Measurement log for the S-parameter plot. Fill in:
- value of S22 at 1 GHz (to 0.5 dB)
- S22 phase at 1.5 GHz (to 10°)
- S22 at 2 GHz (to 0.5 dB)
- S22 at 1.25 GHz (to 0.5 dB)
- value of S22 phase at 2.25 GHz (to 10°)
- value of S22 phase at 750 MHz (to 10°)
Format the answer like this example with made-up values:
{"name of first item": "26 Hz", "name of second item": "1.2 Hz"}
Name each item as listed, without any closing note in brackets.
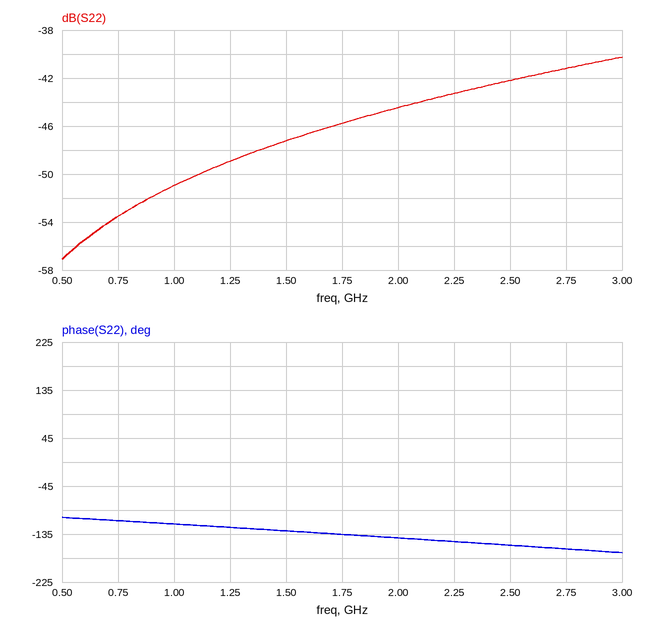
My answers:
{"value of S22 at 1 GHz": "-51.0 dB", "S22 phase at 1.5 GHz": "-130°", "S22 at 2 GHz": "-44.5 dB", "S22 at 1.25 GHz": "-49.0 dB", "value of S22 phase at 2.25 GHz": "-150°", "value of S22 phase at 750 MHz": "-110°"}
